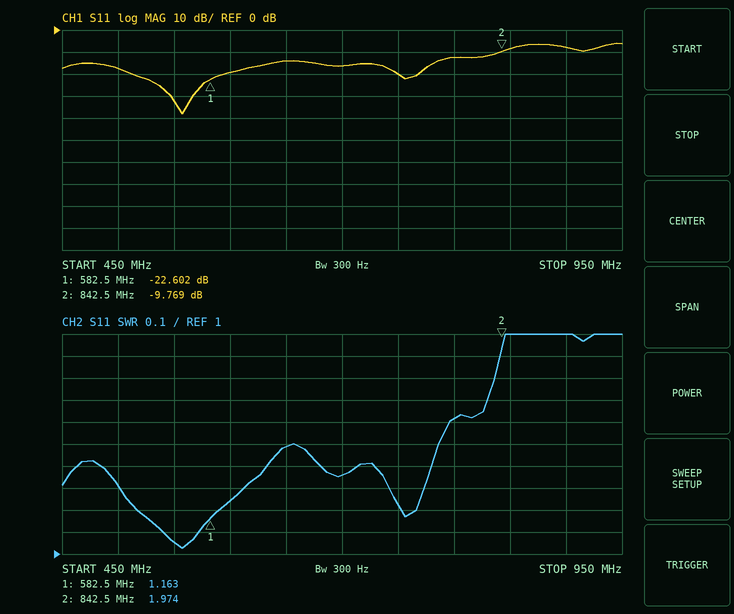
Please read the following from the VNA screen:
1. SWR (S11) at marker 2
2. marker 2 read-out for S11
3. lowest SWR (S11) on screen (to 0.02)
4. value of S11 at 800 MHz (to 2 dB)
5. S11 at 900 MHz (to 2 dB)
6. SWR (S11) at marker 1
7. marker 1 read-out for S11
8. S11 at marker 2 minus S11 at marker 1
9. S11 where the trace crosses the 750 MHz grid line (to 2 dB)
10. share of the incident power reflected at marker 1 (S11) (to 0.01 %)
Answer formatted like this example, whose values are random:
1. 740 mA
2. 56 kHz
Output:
1. 1.974
2. -9.769 dB
3. 1.02
4. -12 dB
5. -8 dB
6. 1.163
7. -22.602 dB
8. 12.833 dB
9. -20 dB
10. 0.55 %
